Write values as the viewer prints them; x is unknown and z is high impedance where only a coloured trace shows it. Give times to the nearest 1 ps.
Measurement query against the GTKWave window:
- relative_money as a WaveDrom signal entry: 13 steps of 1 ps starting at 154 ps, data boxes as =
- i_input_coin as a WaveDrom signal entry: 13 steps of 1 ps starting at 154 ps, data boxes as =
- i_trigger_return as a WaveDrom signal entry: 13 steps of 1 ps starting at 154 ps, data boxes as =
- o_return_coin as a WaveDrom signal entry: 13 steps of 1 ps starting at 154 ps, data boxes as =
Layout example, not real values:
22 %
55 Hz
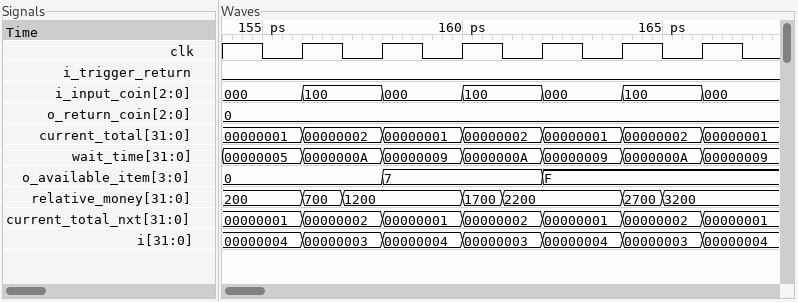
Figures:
{name: 'relative_money', wave: '=.==..==..==.', data: '200 700 1200 1700 2200 2700 3200'}
{name: 'i_input_coin', wave: '=.=.=.=.=.=.=', data: '000 100 000 100 000 100 000'}
{name: 'i_trigger_return', wave: '0............'}
{name: 'o_return_coin', wave: '=............', data: '0'}
